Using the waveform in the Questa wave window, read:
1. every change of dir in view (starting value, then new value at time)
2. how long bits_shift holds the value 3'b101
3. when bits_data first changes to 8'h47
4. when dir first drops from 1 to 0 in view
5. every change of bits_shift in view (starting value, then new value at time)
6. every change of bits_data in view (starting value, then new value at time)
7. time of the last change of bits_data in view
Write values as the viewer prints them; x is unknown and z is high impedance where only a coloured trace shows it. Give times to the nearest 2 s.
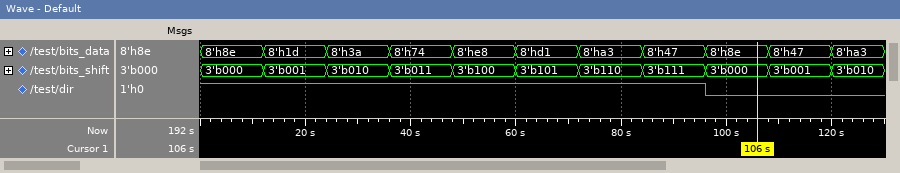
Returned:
1, 0 at 96 s
12 s
84 s
96 s
3'b000, 3'b001 at 12 s, 3'b010 at 24 s, 3'b011 at 36 s, 3'b100 at 48 s, 3'b101 at 60 s, 3'b110 at 72 s, 3'b111 at 84 s, 3'b000 at 96 s, 3'b001 at 108 s, 3'b010 at 120 s
8'h8e, 8'h1d at 12 s, 8'h3a at 24 s, 8'h74 at 36 s, 8'he8 at 48 s, 8'hd1 at 60 s, 8'ha3 at 72 s, 8'h47 at 84 s, 8'h8e at 96 s, 8'h47 at 108 s, 8'ha3 at 120 s
120 s
